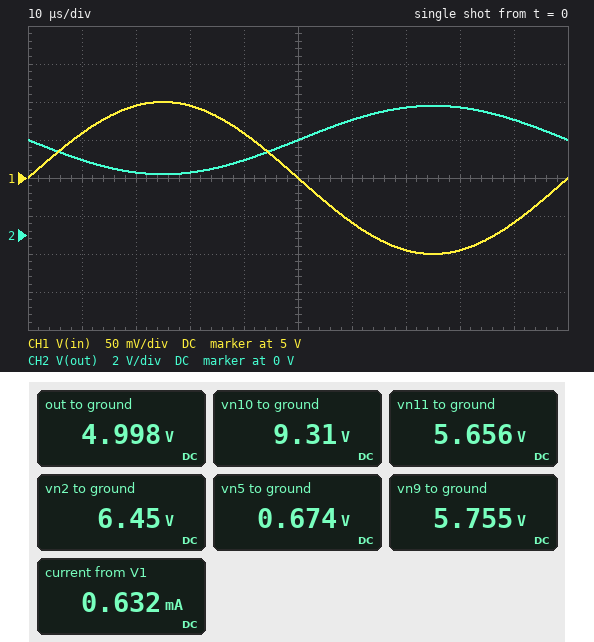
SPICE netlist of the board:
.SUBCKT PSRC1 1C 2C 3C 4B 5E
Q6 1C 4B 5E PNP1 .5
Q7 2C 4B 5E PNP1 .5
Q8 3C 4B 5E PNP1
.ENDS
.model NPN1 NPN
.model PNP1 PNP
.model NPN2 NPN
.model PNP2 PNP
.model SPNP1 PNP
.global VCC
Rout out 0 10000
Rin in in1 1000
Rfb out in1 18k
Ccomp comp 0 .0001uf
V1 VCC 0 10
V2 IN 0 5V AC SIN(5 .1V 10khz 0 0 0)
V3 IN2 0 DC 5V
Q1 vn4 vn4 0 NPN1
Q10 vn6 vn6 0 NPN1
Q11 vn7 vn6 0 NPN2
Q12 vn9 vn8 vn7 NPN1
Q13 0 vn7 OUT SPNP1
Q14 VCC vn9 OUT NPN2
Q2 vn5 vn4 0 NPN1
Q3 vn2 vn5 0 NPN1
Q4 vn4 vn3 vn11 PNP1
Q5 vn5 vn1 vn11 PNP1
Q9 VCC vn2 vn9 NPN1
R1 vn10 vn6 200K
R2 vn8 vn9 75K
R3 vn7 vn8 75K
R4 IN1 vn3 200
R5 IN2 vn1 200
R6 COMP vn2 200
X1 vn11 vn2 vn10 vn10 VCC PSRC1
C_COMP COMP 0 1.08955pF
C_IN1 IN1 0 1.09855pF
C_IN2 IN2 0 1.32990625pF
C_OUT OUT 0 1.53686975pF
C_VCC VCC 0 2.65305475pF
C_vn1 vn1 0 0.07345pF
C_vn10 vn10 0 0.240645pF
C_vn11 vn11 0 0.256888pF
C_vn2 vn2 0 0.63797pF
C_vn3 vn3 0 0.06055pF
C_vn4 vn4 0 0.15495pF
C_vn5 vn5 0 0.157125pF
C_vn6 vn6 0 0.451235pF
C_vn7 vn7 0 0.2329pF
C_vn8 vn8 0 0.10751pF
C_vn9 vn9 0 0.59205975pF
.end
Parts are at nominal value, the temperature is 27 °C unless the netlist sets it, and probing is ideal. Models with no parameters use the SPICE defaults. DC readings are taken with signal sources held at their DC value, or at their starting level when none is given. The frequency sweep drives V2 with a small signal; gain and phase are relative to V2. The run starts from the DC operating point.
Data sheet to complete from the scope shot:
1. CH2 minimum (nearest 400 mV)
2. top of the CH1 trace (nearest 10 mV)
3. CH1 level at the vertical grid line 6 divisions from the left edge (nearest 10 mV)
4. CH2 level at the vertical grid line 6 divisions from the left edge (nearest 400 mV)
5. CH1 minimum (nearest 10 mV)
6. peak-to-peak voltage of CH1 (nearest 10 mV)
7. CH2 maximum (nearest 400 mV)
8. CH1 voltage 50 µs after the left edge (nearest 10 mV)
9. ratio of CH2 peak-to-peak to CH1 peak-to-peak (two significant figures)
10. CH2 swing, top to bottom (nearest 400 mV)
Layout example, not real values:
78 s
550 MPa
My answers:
3.2 V
5.10 V
4.94 V
6.0 V
4.90 V
200 mV
6.8 V
5.00 V
18
3.6 V
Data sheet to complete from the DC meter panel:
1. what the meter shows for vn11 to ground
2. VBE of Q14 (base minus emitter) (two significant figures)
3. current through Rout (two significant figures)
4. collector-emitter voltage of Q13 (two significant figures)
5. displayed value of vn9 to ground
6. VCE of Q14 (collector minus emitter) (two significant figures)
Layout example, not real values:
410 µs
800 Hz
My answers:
5.656 V
760 mV
500 µA
-5.0 V
5.755 V
5.0 V
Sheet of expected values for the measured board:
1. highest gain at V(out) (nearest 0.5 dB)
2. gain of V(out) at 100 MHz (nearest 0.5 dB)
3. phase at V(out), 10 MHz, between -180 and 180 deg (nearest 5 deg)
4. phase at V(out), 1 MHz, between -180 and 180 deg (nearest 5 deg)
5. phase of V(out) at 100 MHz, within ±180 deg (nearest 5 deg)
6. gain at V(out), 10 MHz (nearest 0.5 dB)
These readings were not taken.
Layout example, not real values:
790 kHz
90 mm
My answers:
25.0 dB
-6.5 dB
100 deg
165 deg
30 deg
15.5 dB
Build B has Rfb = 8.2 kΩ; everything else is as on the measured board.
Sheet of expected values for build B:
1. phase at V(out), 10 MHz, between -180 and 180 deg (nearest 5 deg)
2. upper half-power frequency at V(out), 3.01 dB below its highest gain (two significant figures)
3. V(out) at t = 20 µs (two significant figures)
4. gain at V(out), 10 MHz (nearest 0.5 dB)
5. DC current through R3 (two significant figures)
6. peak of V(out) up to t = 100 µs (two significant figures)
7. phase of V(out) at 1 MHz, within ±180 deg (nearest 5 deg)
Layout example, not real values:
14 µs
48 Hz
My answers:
120 deg
7.3 MHz
4.2 V
13.5 dB
9.1 µA
5.8 V
170 deg
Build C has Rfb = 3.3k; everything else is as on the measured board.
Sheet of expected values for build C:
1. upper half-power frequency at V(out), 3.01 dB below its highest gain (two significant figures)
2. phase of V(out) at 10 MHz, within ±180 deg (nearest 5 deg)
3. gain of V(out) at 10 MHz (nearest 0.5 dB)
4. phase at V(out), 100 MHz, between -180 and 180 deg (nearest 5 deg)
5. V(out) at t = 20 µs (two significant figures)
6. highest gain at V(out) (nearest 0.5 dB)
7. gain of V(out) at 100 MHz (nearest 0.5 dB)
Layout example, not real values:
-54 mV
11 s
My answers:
17 MHz
145 deg
9.0 dB
35 deg
4.7 V
10.5 dB
-7.0 dB
